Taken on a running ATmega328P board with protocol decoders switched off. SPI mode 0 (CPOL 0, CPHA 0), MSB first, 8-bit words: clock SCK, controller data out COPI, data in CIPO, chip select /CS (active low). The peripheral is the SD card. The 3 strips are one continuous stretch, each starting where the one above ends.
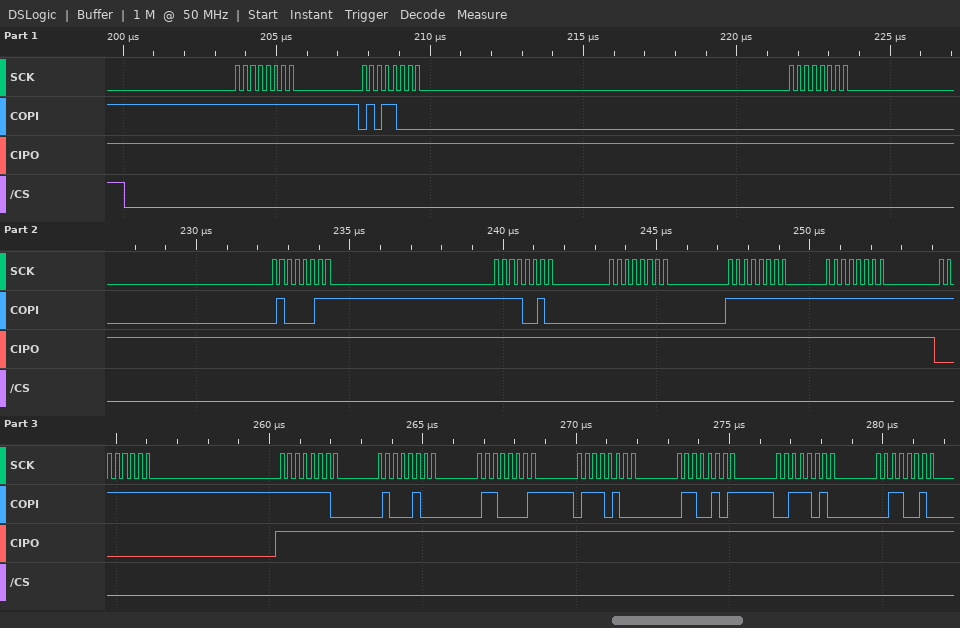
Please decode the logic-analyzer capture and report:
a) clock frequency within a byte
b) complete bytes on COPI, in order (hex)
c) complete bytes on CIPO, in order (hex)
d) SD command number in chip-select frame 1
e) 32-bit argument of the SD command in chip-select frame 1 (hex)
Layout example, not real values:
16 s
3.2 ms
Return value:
4 MHz
FF 58 00 43 F2 00 FF FF FF FE 44 61 74 65 3A 32
FF FF FF FF FF FF FF FF 00 FF FF FF FF FF FF FF
CMD24
0x0043F200
